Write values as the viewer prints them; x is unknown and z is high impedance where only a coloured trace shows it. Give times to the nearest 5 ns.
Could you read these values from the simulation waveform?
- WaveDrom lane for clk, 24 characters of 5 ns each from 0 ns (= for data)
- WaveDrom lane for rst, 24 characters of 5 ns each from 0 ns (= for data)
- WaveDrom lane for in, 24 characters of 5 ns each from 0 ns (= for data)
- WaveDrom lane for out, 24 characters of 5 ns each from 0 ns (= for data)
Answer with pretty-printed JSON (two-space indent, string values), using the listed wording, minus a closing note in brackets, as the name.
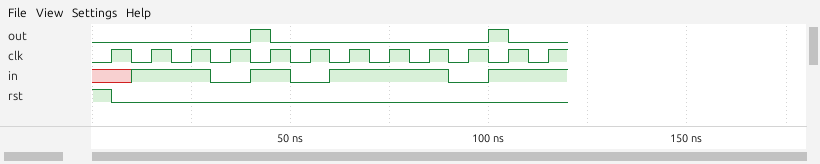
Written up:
{
  "WaveDrom lane for clk, 24 characters of 5 ns each from 0 ns": "{name: 'clk', wave: '010101010101010101010101'}",
  "WaveDrom lane for rst, 24 characters of 5 ns each from 0 ns": "{name: 'rst', wave: '10......................'}",
  "WaveDrom lane for in, 24 characters of 5 ns each from 0 ns": "{name: 'in', wave: 'x.1...0.1.0.1.....0.1...'}",
  "WaveDrom lane for out, 24 characters of 5 ns each from 0 ns": "{name: 'out', wave: '0.......10..........10..'}"
}
